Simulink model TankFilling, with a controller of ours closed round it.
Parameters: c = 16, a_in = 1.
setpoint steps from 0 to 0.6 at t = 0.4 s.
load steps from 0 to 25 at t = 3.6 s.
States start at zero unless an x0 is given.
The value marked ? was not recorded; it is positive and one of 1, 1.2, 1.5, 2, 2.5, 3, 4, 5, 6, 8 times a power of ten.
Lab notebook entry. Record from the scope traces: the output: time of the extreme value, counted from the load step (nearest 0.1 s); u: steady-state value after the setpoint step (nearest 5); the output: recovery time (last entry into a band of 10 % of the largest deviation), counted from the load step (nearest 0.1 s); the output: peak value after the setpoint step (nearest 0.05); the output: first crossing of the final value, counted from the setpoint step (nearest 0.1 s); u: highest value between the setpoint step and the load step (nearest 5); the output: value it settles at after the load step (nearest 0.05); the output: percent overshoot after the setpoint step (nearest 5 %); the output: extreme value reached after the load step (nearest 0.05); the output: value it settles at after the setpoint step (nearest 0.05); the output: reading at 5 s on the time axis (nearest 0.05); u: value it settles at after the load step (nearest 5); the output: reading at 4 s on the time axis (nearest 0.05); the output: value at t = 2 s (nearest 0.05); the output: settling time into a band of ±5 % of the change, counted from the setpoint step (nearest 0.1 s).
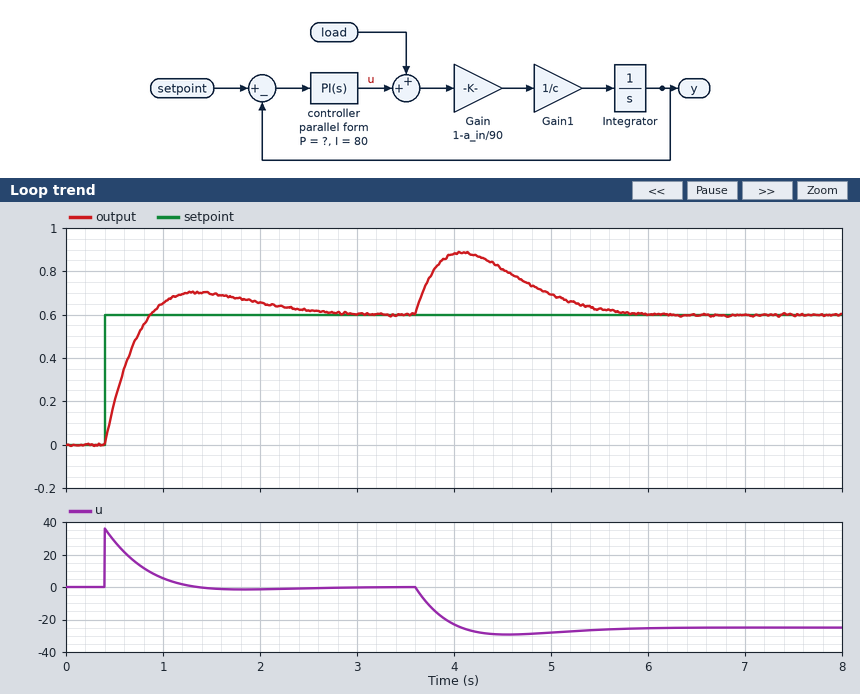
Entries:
0.5 s
0
1.9 s
0.70
0.5 s
35
0.60
15 %
0.90
0.60
0.70
-25
0.90
0.65
1.9 s
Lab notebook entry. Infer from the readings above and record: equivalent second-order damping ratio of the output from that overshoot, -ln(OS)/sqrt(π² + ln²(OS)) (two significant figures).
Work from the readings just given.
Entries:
0.52
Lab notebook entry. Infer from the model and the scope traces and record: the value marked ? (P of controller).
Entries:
60
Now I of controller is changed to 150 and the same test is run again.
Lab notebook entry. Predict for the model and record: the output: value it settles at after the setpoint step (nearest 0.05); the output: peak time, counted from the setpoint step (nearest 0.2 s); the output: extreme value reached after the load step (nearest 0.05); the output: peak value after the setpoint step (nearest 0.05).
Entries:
0.60
0.8 s
0.85
0.75
